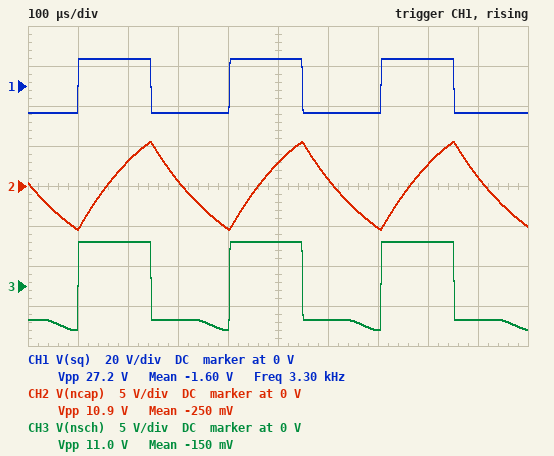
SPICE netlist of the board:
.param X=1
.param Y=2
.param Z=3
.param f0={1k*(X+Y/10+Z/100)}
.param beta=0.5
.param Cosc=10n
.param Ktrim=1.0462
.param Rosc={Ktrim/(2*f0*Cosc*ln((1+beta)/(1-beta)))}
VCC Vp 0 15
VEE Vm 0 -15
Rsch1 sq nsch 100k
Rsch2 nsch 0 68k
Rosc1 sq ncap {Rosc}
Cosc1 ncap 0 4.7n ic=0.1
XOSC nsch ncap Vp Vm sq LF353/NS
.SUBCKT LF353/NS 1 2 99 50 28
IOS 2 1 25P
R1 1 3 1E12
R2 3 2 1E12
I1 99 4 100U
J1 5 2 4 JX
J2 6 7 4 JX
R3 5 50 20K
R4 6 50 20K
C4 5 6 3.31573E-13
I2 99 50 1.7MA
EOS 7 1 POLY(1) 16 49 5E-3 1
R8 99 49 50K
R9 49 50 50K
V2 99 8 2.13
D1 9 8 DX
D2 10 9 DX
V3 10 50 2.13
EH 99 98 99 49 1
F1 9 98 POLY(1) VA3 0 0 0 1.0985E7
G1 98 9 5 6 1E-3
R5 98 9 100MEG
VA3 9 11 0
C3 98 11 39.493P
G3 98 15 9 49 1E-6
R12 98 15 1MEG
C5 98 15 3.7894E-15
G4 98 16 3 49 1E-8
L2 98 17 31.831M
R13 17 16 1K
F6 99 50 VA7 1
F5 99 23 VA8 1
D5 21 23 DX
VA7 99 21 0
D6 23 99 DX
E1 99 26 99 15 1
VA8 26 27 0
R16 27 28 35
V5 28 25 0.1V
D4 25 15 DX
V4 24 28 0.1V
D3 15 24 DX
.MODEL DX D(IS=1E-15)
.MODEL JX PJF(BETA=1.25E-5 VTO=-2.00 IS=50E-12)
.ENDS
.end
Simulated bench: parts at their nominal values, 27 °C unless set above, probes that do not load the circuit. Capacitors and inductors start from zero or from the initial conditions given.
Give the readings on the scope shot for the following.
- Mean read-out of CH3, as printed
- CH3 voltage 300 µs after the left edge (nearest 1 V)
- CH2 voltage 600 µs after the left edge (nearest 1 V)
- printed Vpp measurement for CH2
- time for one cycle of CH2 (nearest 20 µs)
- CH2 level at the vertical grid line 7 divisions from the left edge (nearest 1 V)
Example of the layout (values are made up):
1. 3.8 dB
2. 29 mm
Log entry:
1. -150 mV
2. -4 V
3. 1 V
4. 10.9 V
5. 300 µs
6. -5 V
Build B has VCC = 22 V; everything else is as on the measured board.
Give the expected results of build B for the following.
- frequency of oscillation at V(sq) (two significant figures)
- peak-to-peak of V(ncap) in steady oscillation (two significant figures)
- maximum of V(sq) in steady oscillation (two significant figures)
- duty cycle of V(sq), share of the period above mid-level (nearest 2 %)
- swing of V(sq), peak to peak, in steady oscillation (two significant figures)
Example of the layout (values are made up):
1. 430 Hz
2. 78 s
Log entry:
1. 3.2 kHz
2. 14 V
3. 21 V
4. 42 %
5. 34 V
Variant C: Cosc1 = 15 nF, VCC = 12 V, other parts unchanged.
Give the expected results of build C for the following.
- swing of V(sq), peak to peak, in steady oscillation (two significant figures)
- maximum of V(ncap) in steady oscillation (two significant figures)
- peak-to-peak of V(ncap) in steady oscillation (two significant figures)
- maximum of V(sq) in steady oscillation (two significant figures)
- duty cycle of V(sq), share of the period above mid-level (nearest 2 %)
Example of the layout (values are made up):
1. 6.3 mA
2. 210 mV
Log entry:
1. 24 V
2. 4.2 V
3. 9.7 V
4. 11 V
5. 52 %
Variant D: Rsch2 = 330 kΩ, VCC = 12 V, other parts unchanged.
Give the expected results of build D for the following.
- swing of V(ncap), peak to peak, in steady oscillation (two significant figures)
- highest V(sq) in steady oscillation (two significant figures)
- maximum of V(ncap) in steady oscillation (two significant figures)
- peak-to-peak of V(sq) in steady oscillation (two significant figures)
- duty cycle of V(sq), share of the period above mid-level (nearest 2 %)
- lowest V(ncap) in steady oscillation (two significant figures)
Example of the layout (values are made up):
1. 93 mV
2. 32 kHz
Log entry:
1. 18 V
2. 11 V
3. 8.0 V
4. 24 V
5. 50 %
6. -10 V
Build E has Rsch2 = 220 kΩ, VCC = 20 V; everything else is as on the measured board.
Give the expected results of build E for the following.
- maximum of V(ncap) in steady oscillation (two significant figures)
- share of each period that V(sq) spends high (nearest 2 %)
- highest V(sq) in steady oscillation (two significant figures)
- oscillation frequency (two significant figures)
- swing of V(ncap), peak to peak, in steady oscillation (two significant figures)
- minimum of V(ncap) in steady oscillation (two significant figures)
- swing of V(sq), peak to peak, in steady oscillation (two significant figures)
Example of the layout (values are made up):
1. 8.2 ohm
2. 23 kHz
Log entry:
1. 13 V
2. 44 %
3. 19 V
4. 1.7 kHz
5. 22 V
6. -9.3 V
7. 32 V
